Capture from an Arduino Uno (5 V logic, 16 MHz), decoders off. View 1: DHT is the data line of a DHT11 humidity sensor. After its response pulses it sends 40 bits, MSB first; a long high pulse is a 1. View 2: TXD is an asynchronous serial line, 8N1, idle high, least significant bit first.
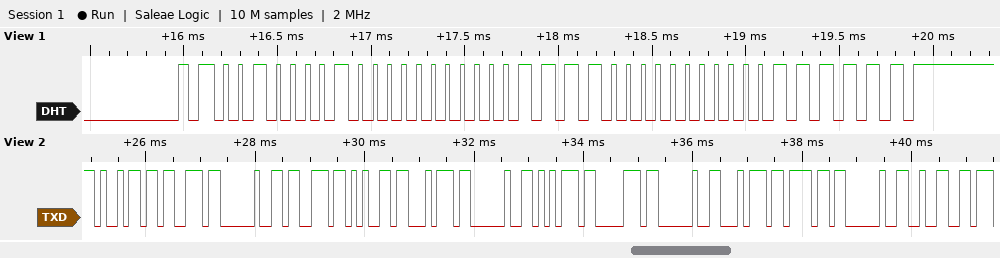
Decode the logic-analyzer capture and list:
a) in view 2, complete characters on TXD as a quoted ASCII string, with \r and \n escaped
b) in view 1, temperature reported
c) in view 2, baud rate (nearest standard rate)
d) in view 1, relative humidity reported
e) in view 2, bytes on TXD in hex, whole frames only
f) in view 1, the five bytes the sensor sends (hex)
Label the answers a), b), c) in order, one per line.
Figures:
a) "is set up to 2"
b) 30.0 °C
c) 9600 baud
d) 33 %
e) 69 73 20 73 65 74 20 75 70 20 74 6F 20 32
f) 21 00 1E 00 3F
